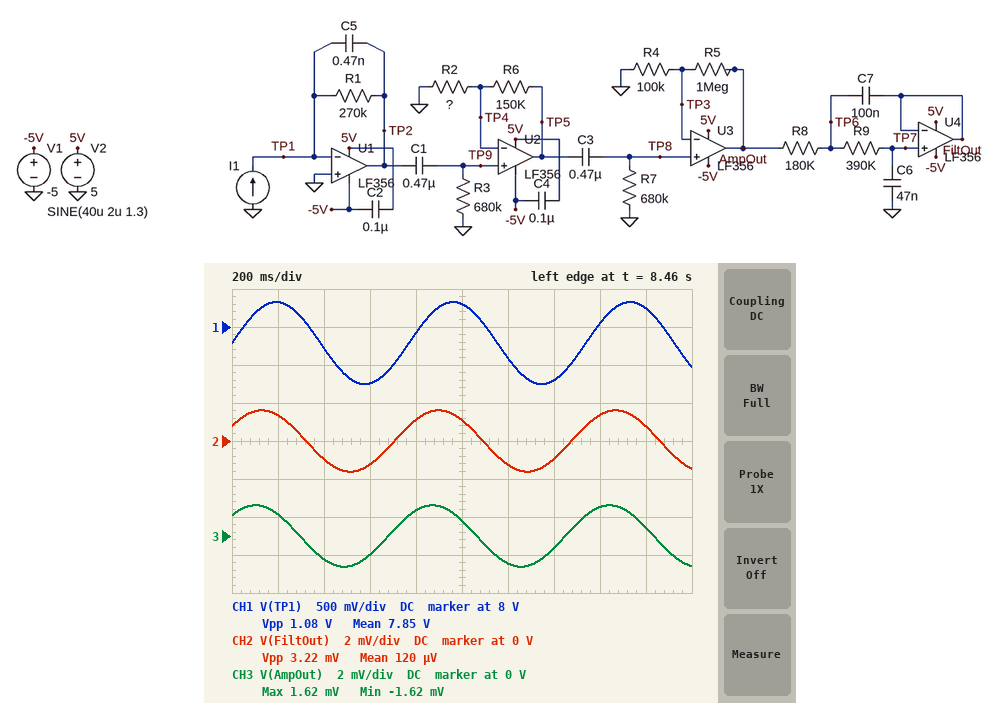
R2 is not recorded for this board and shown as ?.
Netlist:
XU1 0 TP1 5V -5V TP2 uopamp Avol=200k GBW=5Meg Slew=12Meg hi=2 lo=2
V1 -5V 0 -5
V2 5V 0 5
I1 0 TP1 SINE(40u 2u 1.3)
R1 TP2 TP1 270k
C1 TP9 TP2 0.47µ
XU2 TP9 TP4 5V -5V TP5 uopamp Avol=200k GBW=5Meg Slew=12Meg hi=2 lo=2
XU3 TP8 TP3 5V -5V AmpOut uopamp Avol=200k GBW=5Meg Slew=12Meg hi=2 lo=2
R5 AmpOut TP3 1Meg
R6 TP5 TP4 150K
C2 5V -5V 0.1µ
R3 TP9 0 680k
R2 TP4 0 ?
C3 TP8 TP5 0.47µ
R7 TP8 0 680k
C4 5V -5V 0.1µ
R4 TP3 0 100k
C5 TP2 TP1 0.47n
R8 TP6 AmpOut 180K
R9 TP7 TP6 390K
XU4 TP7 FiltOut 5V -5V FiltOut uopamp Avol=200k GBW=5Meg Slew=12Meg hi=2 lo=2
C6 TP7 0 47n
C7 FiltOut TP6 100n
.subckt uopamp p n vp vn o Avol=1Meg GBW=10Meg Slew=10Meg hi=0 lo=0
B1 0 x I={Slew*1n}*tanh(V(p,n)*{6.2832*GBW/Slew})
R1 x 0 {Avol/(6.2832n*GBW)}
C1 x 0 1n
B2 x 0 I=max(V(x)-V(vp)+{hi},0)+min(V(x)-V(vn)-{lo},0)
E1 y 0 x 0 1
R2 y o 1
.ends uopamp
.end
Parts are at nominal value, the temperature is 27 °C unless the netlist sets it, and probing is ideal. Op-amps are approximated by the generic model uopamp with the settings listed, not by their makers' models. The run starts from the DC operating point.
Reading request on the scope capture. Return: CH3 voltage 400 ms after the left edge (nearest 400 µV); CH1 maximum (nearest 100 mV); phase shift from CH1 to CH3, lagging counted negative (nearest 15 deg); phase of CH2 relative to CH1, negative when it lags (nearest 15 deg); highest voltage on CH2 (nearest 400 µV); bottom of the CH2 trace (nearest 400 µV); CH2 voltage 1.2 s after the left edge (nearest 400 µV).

-1.2 mV
8.3 V
45 deg
30 deg
1.6 mV
-1.6 mV
-1.2 mV
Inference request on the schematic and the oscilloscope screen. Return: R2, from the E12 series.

1.8 kΩ
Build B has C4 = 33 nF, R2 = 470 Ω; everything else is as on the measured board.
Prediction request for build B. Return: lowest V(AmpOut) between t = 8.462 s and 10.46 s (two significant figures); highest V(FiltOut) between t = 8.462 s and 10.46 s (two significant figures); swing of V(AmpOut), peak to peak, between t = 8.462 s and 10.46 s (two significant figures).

-6.1 mV
6.1 mV
12 mV
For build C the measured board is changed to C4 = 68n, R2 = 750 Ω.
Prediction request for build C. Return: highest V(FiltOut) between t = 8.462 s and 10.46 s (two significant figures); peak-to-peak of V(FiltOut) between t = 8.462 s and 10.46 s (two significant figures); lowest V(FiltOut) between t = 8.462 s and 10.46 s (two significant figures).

3.8 mV
7.7 mV
-3.8 mV
